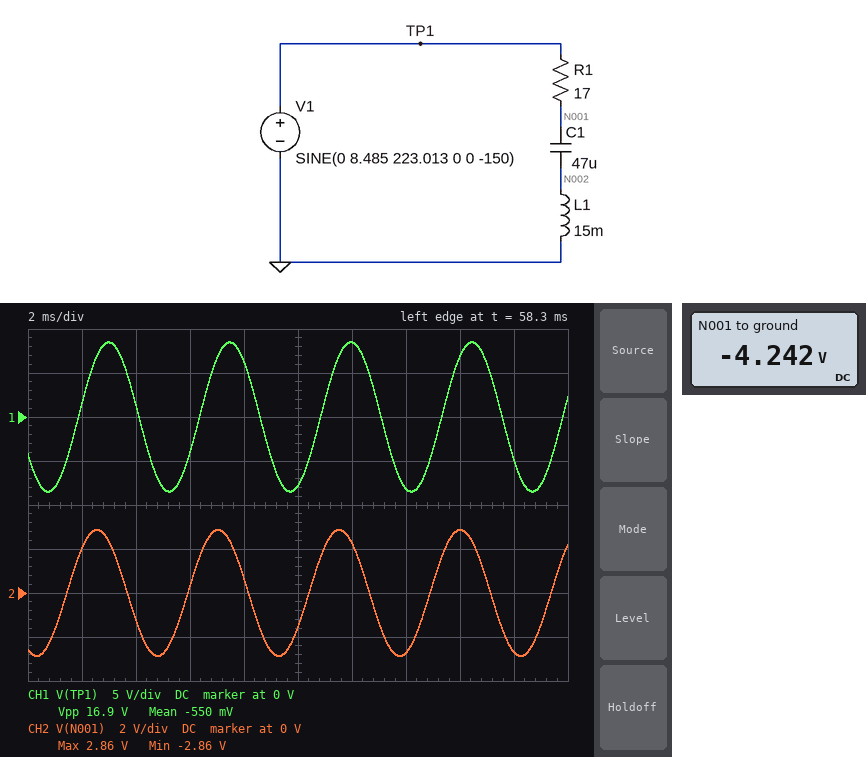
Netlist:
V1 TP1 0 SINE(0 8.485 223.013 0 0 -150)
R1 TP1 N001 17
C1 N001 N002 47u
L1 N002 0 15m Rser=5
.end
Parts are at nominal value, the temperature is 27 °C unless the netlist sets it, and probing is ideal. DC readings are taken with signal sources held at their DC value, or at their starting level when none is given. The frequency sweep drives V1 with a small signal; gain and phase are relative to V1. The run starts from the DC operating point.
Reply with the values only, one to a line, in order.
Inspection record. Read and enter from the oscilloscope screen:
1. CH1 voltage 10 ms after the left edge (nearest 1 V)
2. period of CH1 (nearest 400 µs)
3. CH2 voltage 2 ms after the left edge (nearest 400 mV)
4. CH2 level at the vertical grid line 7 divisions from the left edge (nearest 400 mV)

-8 V
4.4 ms
2.0 V
-2.8 V
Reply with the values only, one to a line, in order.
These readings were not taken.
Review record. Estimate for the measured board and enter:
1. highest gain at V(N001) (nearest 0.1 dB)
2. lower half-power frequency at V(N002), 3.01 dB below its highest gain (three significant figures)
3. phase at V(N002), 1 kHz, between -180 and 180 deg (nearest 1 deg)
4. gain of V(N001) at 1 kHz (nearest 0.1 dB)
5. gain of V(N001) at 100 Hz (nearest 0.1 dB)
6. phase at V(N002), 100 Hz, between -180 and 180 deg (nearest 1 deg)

0 dB
167 Hz
11 deg
-0.2 dB
-2.4 dB
110 deg
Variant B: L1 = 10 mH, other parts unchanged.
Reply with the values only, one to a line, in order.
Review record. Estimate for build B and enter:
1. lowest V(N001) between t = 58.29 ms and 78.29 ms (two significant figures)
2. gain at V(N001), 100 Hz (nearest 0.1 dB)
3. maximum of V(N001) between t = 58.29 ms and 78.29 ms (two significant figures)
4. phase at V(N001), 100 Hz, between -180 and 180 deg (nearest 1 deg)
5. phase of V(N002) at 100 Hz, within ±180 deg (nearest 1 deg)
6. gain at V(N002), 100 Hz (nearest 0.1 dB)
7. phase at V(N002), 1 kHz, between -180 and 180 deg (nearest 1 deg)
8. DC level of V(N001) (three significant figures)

-2.0 V
-2.0 dB
2.0 V
-28 deg
103 deg
-12.9 dB
16 deg
-4.24 V
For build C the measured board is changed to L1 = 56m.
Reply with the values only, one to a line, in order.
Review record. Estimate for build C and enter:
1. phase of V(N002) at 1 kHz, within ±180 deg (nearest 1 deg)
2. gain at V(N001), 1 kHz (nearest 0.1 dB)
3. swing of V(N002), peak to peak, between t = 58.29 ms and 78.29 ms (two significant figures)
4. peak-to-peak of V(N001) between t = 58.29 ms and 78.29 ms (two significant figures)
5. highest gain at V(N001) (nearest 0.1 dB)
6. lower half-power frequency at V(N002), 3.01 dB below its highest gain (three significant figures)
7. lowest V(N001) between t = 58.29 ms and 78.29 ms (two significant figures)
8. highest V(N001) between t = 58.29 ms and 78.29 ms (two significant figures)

3 deg
0 dB
20 V
16 V
0 dB
82.7 Hz
-8.0 V
8.0 V
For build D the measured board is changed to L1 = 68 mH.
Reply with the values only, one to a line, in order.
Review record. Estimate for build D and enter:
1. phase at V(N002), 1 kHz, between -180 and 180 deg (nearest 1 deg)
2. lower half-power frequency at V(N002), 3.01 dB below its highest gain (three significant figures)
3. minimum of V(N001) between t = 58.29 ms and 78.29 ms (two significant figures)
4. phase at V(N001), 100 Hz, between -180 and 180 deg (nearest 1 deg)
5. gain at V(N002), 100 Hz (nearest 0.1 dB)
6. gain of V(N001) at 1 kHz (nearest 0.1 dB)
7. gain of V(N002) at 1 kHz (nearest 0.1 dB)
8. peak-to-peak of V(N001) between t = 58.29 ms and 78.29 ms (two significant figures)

2 deg
75.5 Hz
-8.2 V
39 deg
5.2 dB
0 dB
0.1 dB
16 V
